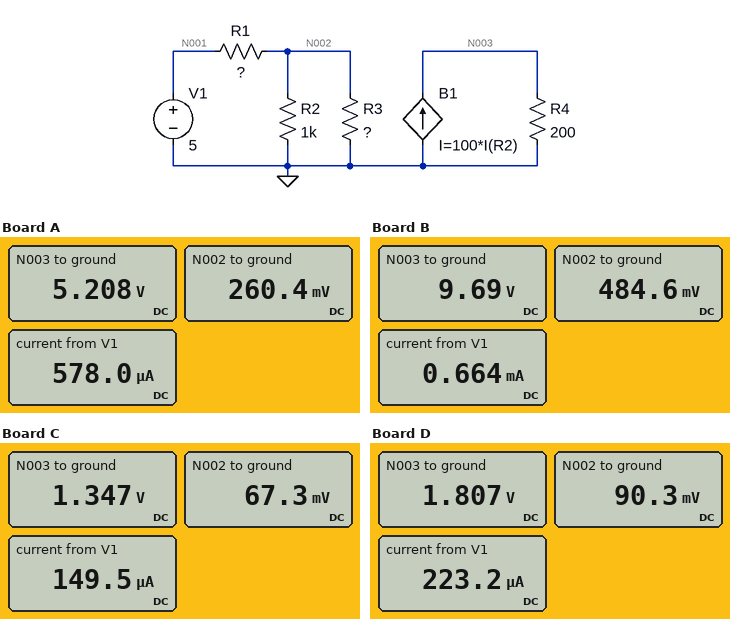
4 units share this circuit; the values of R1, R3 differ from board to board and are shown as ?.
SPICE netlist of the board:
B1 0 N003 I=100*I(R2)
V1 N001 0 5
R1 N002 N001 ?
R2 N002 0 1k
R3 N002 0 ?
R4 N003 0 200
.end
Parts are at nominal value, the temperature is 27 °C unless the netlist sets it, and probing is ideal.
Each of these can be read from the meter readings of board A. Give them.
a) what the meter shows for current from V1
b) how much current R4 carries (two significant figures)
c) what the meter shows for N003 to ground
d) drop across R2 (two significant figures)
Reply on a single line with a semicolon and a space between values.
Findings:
578.0 µA; 26 mA; 5.208 V; 260 mV
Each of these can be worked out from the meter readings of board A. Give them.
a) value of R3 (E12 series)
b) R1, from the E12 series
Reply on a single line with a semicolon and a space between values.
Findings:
820 Ω; 8.2 kΩ
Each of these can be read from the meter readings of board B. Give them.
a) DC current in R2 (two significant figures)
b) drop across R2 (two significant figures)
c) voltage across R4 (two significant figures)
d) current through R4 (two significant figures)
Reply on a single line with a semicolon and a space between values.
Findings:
480 µA; 480 mV; 9.7 V; 48 mA
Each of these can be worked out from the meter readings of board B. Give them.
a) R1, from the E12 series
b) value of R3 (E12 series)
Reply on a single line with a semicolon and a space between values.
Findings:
6.8 kΩ; 2.7 kΩ
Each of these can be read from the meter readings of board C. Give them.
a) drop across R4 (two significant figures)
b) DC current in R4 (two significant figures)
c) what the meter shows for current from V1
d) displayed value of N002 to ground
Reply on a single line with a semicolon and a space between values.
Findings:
1.3 V; 6.7 mA; 149.5 µA; 67.3 mV
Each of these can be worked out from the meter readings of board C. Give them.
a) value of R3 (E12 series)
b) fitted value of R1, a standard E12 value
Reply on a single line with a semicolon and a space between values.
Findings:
820 Ω; 33 kΩ
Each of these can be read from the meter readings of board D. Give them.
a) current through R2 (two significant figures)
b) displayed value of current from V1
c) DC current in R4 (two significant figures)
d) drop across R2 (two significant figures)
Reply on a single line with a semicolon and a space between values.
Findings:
90 µA; 223.2 µA; 9.0 mA; 90 mV
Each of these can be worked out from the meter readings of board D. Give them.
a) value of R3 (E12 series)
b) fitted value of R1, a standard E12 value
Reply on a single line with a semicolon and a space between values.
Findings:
680 Ω; 22 kΩ
